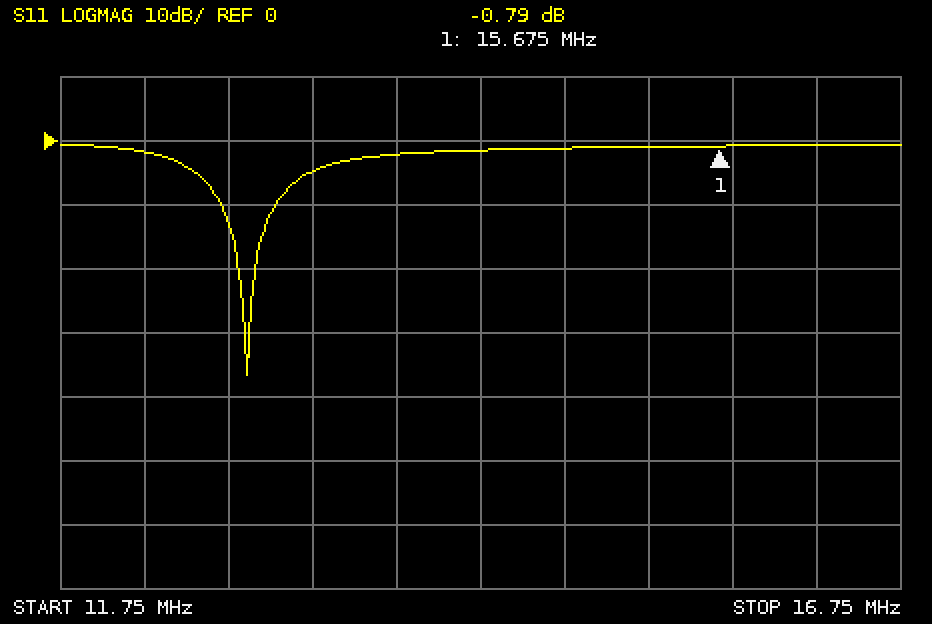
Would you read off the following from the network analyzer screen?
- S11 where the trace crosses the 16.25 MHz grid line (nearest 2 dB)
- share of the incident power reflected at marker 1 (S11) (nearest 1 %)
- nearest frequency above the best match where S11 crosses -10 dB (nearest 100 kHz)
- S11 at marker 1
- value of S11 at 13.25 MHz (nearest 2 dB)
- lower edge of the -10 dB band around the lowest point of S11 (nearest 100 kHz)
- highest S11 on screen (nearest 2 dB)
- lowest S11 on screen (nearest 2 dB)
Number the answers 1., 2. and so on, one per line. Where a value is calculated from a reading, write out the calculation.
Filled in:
1. 0 dB
2. 10^(-0.79/10) ≈ 83 %
3. 13.0 MHz
4. -0.79 dB
5. -4 dB
6. 12.7 MHz
7. 0 dB
8. -36 dB
